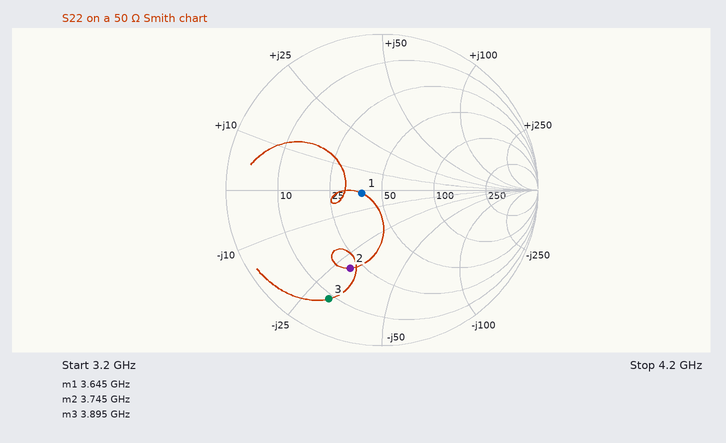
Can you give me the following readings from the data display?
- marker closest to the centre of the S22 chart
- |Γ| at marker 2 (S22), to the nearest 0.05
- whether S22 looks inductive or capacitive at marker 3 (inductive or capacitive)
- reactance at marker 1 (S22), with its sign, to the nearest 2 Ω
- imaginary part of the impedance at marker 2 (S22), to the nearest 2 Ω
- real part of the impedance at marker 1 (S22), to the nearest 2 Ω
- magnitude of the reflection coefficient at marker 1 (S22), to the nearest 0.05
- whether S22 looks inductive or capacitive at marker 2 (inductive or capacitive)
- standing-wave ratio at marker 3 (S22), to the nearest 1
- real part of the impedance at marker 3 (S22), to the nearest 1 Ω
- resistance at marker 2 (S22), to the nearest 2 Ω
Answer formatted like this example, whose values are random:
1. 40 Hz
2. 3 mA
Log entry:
1. marker 1
2. 0.55
3. capacitive
4. -2 Ω
5. -30 Ω
6. 38 Ω
7. 0.15
8. capacitive
9. 8
10. 9 Ω
11. 20 Ω
